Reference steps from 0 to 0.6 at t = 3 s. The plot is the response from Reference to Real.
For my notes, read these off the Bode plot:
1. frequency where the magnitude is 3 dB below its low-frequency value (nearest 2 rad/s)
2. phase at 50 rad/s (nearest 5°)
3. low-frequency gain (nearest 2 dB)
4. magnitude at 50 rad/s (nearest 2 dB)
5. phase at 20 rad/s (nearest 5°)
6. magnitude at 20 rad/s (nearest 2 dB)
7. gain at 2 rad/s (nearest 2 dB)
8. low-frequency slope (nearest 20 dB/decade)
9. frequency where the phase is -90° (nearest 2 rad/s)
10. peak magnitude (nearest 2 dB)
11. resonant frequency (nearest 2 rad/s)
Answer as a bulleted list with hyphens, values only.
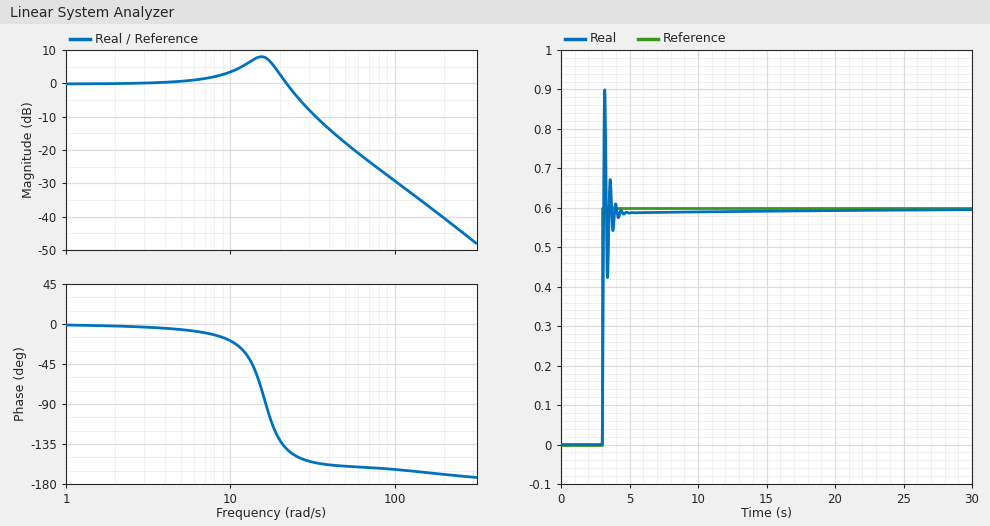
- 24 rad/s
- -160°
- 0 dB
- -18 dB
- -130°
- 2 dB
- 0 dB
- 0 dB/decade
- 16 rad/s
- 8 dB
- 16 rad/s
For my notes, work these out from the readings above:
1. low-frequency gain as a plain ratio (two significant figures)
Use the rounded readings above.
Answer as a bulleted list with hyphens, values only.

- 1.0
